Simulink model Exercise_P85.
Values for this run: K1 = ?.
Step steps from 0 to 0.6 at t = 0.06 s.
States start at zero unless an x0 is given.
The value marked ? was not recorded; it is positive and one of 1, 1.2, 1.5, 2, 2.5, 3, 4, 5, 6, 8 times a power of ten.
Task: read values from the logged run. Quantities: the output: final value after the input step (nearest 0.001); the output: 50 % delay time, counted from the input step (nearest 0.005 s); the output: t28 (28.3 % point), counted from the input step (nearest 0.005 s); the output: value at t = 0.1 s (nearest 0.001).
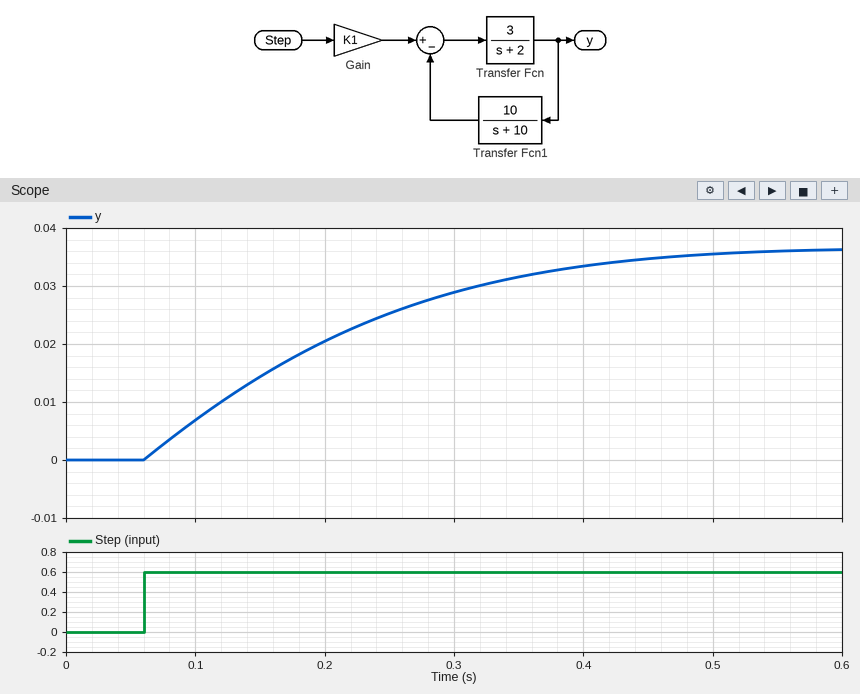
0.036
0.120 s
0.060 s
0.007
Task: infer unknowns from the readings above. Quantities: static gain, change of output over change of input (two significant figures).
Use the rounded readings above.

0.060
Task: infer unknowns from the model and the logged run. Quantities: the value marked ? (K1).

0.1
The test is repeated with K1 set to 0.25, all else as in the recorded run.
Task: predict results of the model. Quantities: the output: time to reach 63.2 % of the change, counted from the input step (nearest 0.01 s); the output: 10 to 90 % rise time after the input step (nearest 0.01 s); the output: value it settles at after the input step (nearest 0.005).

0.16 s
0.29 s
0.090
